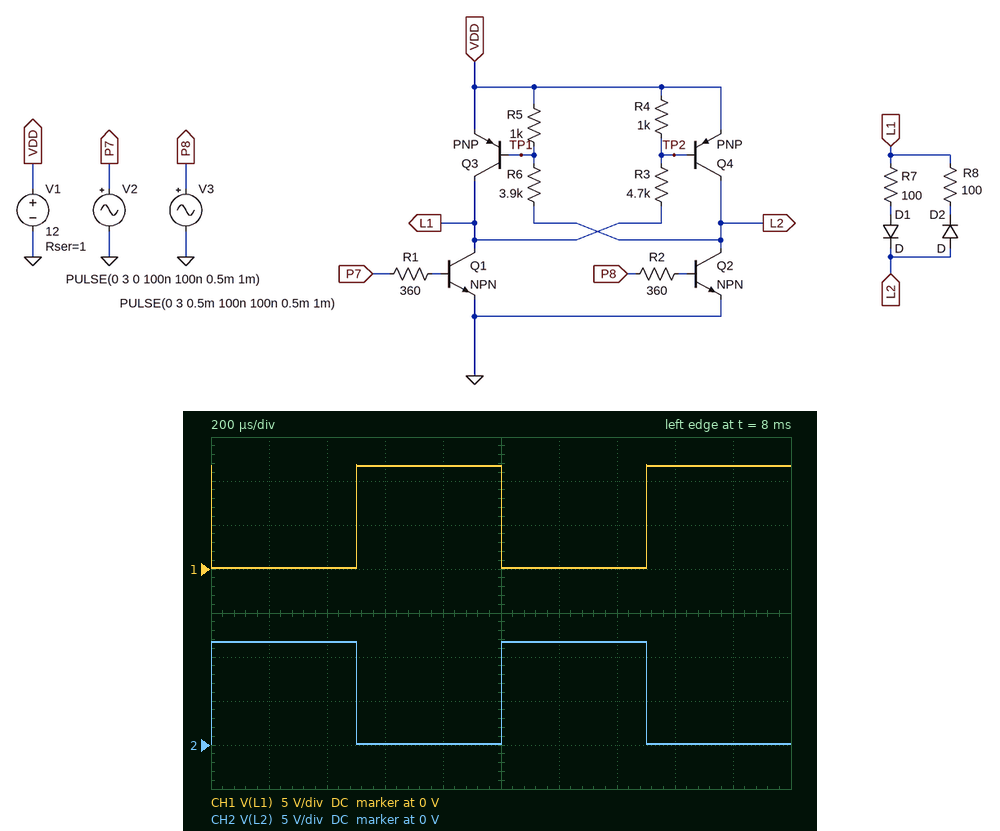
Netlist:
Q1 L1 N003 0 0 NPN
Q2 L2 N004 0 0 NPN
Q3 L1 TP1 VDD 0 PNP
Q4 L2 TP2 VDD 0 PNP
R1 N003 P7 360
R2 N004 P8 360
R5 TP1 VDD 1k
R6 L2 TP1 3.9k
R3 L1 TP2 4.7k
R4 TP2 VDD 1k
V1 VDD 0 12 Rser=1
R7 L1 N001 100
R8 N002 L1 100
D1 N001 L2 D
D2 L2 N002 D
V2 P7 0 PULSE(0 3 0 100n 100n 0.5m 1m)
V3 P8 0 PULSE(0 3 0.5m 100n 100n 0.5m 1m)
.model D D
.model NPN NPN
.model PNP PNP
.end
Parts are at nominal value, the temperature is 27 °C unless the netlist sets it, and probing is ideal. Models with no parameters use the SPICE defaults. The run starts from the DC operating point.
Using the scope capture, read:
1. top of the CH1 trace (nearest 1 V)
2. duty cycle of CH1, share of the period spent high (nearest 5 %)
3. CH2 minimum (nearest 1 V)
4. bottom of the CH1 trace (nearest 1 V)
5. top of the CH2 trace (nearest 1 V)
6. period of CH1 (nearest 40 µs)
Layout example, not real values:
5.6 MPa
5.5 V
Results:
12 V
50 %
0 V
0 V
12 V
1.00 ms
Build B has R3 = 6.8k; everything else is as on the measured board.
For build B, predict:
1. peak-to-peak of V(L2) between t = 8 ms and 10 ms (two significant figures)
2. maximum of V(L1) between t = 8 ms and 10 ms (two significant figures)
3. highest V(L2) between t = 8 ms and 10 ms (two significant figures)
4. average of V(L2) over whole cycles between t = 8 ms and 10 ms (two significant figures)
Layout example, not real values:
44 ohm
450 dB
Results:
8.1 V
12 V
8.2 V
4.1 V
